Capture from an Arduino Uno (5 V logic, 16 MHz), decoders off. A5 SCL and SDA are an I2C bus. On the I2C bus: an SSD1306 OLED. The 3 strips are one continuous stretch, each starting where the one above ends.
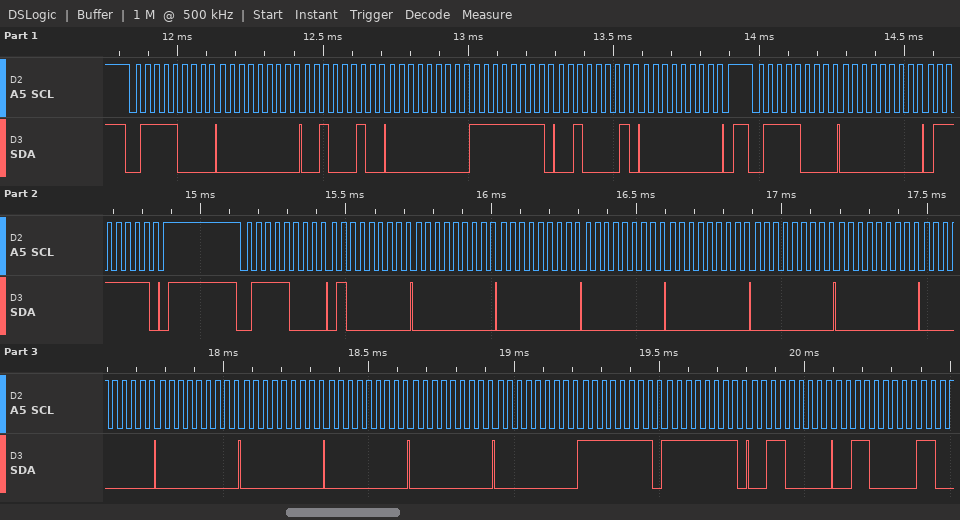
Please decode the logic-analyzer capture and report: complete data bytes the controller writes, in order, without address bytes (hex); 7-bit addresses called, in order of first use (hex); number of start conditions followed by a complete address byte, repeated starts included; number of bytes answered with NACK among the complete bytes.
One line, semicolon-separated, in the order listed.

00 22 00 FF 21 00 00 7F 40 00 00 00 00 00 00 00 00 00 00 00 00 FF FF 30 30; 0x3C; 3; 0
